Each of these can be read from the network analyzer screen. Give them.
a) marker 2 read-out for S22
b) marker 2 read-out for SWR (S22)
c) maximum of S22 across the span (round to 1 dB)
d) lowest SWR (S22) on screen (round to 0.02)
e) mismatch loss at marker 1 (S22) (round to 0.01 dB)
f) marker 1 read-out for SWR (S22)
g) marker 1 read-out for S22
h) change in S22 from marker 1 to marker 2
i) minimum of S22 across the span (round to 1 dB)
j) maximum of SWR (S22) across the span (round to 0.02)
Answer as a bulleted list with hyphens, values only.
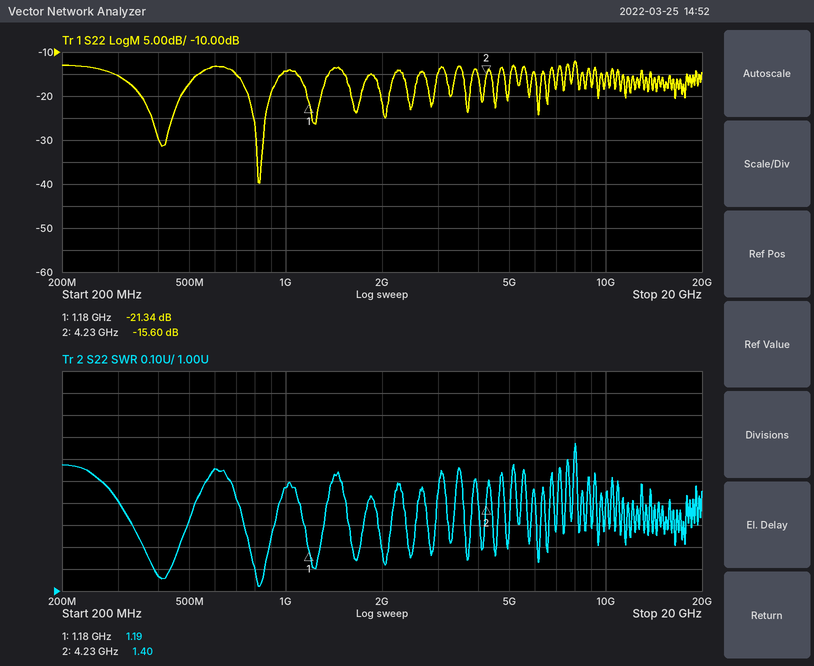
- -15.60 dB
- 1.40
- -12 dB
- 1.02
- 0.03 dB
- 1.19
- -21.34 dB
- 5.74 dB
- -40 dB
- 1.68
